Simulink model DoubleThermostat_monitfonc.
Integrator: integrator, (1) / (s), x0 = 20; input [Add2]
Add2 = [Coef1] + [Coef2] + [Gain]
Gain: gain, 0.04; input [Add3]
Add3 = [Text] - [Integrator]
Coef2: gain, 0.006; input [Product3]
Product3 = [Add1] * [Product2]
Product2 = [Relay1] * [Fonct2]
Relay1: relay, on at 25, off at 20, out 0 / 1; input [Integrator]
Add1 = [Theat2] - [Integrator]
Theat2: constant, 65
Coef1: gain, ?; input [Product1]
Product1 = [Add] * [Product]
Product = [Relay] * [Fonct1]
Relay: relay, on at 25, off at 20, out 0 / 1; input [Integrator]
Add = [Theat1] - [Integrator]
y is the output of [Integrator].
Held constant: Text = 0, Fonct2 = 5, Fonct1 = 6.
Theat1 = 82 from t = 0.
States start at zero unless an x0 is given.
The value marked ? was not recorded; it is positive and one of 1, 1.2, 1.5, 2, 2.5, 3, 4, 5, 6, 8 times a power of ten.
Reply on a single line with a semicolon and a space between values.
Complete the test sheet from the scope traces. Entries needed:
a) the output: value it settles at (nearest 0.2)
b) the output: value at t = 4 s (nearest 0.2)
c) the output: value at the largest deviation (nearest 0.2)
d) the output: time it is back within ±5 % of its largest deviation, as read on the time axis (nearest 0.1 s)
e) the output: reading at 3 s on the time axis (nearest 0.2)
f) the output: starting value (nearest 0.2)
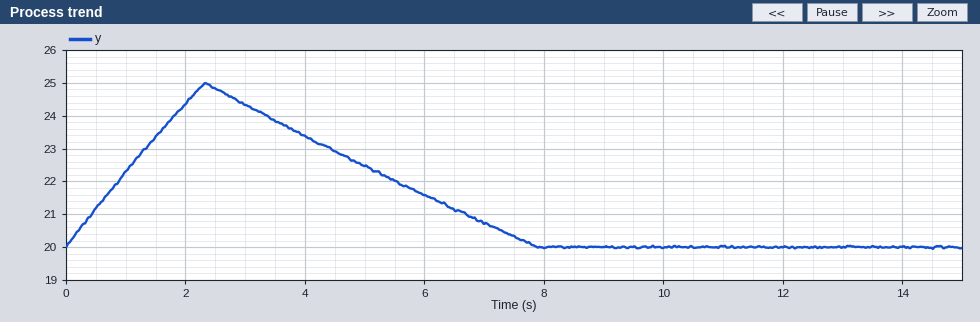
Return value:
20.0; 23.4; 25.0; 7.6 s; 24.4; 20.0
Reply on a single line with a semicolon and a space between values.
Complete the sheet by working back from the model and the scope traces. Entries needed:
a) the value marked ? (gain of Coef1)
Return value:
0.005
